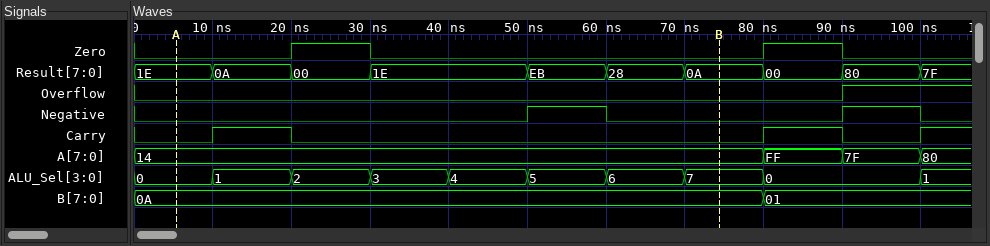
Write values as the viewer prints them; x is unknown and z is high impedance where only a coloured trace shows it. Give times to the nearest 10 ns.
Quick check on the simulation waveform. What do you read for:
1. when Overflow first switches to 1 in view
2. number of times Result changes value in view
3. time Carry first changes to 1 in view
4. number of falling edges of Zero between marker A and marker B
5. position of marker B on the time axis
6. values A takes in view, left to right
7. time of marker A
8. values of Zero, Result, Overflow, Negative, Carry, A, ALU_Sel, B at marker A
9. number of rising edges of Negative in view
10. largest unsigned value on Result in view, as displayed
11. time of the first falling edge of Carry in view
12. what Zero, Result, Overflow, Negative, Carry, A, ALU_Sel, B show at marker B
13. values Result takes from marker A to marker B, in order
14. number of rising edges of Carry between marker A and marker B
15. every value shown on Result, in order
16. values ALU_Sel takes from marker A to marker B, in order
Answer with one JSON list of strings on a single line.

["90 ns", "9", "10 ns", "1", "70 ns", "14, FF, 7F, 80", "10 ns", "Zero=0, Result=1E, Overflow=0, Negative=0, Carry=0, A=14, ALU_Sel=0, B=0A", "2", "EB", "20 ns", "Zero=0, Result=0A, Overflow=0, Negative=0, Carry=0, A=14, ALU_Sel=7, B=0A", "1E, 0A, 00, 1E, EB, 28, 0A", "1", "1E, 0A, 00, 1E, EB, 28, 0A, 00, 80, 7F", "0, 1, 2, 3, 4, 5, 6, 7"]
